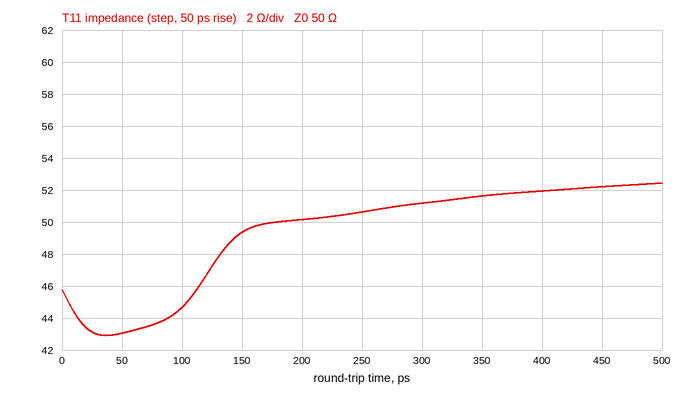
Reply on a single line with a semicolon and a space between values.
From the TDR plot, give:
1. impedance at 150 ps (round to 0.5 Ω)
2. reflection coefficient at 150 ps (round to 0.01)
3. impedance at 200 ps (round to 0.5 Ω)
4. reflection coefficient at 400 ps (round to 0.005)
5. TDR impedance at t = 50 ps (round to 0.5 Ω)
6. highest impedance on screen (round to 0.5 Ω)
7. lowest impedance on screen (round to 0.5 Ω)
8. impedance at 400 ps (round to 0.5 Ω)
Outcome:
49.5 Ω; -0.01; 50.0 Ω; +0.020; 43.0 Ω; 52.5 Ω; 43.0 Ω; 52.0 Ω
